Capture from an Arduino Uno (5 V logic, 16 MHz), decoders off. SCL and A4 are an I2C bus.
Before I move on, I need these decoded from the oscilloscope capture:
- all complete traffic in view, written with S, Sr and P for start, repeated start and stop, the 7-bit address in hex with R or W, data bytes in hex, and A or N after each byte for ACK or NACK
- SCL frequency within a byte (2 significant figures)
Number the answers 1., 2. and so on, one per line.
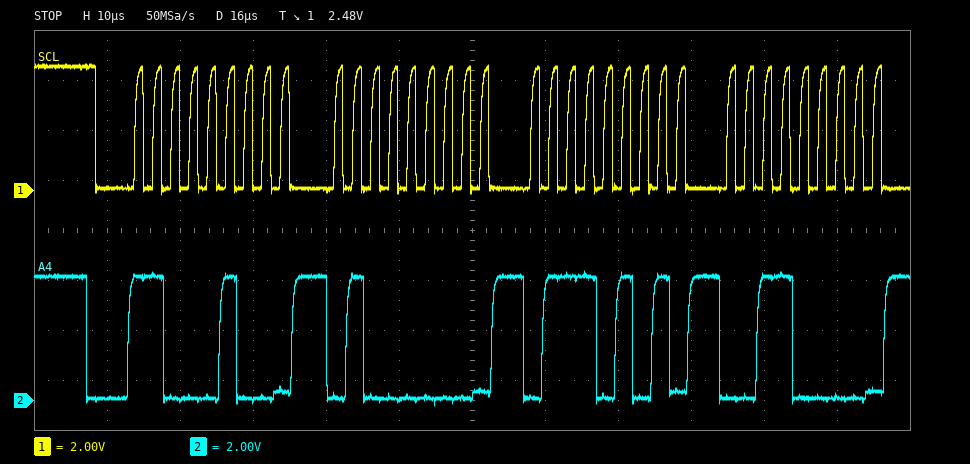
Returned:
1. S 62W A 40 A 75 A 30 A
2. 400 kHz
